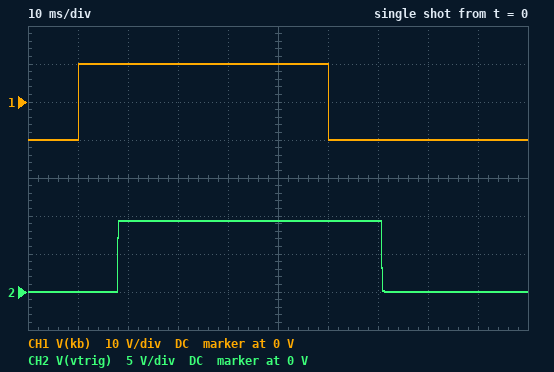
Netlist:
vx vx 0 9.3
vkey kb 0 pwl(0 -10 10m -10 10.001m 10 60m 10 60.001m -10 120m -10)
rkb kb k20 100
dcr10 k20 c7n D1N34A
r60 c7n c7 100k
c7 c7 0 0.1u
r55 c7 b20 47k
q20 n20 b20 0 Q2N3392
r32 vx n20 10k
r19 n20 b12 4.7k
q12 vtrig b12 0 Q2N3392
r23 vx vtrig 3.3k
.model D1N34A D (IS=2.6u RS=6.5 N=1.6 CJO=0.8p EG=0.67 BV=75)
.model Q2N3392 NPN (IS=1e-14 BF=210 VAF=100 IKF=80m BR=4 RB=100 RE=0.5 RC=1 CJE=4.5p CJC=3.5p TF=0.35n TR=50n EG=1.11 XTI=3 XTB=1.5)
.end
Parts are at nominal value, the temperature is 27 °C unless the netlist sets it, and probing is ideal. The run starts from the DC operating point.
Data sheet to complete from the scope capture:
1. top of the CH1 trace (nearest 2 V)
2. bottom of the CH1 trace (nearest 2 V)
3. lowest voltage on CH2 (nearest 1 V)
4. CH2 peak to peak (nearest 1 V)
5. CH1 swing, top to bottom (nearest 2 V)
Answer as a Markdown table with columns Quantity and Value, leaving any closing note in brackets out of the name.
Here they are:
| Quantity | Value |
|---|---|
| top of the CH1 trace | 10 V |
| bottom of the CH1 trace | -10 V |
| lowest voltage on CH2 | 0 V |
| CH2 peak to peak | 9 V |
| CH1 swing, top to bottom | 20 V |
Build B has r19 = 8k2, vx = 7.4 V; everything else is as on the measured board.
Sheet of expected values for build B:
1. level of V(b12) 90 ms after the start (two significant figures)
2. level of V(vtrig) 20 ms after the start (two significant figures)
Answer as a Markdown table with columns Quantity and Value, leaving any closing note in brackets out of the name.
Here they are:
| Quantity | Value |
|---|---|
| level of V(b12) 90 ms after the start | 730 mV |
| level of V(vtrig) 20 ms after the start | 7.4 V |
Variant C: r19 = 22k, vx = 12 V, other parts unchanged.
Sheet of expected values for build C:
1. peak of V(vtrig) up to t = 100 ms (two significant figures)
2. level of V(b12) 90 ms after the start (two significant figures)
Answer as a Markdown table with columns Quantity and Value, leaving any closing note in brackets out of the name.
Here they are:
| Quantity | Value |
|---|---|
| peak of V(vtrig) up to t = 100 ms | 12 V |
| level of V(b12) 90 ms after the start | 740 mV |
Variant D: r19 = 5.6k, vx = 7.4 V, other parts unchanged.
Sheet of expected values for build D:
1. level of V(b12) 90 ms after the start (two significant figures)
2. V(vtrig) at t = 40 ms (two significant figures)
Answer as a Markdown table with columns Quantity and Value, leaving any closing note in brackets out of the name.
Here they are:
| Quantity | Value |
|---|---|
| level of V(b12) 90 ms after the start | 740 mV |
| V(vtrig) at t = 40 ms | 7.4 V |
